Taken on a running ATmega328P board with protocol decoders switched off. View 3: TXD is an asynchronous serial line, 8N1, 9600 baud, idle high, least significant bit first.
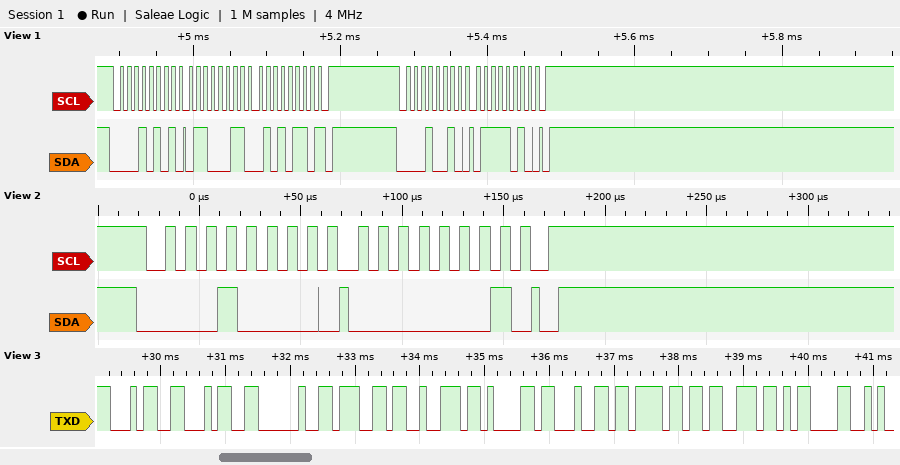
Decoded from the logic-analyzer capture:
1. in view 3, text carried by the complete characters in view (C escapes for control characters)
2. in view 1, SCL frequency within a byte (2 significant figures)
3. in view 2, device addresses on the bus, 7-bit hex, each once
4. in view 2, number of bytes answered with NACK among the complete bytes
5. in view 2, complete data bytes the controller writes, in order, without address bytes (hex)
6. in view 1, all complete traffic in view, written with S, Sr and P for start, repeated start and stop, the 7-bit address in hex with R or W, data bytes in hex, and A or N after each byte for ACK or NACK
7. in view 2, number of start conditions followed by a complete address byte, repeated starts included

"44 grados\r"
100 kHz
0x08
0
01
S 0AR A 63 A 56 N P S 09W A 7A A P
1
